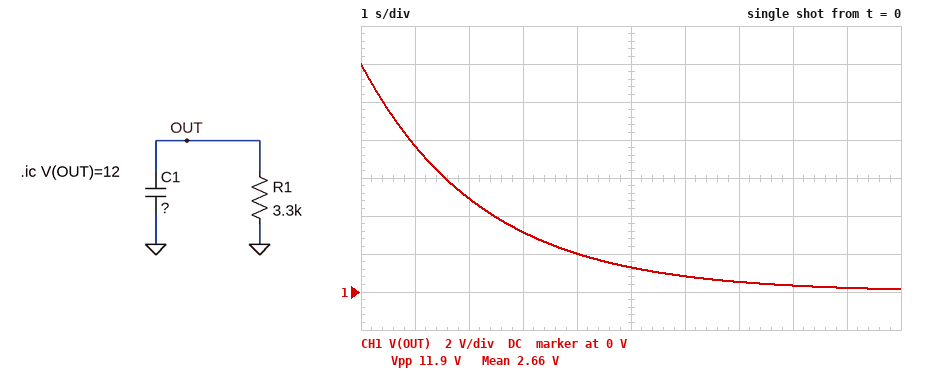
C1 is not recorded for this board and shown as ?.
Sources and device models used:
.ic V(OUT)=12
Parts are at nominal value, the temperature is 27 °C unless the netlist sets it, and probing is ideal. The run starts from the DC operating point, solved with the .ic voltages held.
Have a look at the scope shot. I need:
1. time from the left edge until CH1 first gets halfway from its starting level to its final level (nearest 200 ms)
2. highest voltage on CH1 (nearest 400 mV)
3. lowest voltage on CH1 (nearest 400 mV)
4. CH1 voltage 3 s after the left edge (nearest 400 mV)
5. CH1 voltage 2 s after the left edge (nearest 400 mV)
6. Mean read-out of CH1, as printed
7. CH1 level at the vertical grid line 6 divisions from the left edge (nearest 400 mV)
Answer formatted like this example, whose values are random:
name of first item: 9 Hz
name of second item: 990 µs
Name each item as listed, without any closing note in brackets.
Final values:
time from the left edge until CH1 first gets halfway from its starting level to its final level: 1.6 s
highest voltage on CH1: 12.0 V
lowest voltage on CH1: 0 V
CH1 voltage 3 s after the left edge: 3.2 V
CH1 voltage 2 s after the left edge: 4.8 V
Mean read-out of CH1, as printed: 2.66 V
CH1 level at the vertical grid line 6 divisions from the left edge: 800 mV
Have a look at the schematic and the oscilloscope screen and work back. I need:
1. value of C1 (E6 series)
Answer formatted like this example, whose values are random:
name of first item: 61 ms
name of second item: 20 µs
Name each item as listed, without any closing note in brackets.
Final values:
value of C1: 680 µF
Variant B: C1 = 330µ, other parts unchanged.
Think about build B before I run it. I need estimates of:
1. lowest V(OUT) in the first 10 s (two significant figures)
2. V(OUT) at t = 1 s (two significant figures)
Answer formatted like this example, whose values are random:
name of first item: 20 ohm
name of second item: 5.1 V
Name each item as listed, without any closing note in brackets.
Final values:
lowest V(OUT) in the first 10 s: 1.2 mV
V(OUT) at t = 1 s: 4.8 V
